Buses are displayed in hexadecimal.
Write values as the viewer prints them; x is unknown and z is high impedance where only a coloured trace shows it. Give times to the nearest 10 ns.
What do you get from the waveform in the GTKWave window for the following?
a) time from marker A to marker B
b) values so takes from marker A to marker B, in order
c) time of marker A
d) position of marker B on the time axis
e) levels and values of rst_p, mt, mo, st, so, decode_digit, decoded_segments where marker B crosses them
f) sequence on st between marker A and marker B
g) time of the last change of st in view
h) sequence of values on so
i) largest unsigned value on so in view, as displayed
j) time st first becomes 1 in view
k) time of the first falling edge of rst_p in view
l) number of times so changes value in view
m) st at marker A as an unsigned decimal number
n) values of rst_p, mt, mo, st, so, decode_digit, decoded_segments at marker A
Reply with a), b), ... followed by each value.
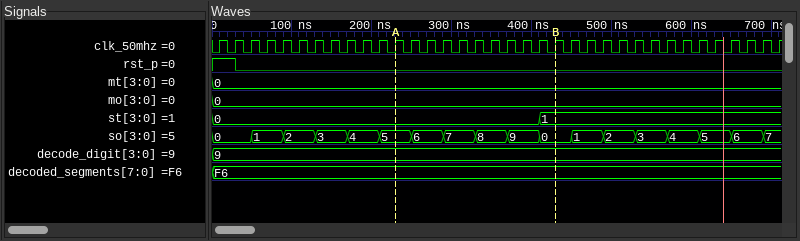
a) 200 ns
b) 5, 6, 7, 8, 9, 0
c) 230 ns
d) 430 ns
e) rst_p=0, mt=0, mo=0, st=1, so=0, decode_digit=9, decoded_segments=F6
f) 0, 1
g) 410 ns
h) 0, 1, 2, 3, 4, 5, 6, 7, 8, 9, 0, 1, 2, 3, 4, 5, 6, 7
i) 9
j) 410 ns
k) 30 ns
l) 17
m) 0
n) rst_p=0, mt=0, mo=0, st=0, so=5, decode_digit=9, decoded_segments=F6
